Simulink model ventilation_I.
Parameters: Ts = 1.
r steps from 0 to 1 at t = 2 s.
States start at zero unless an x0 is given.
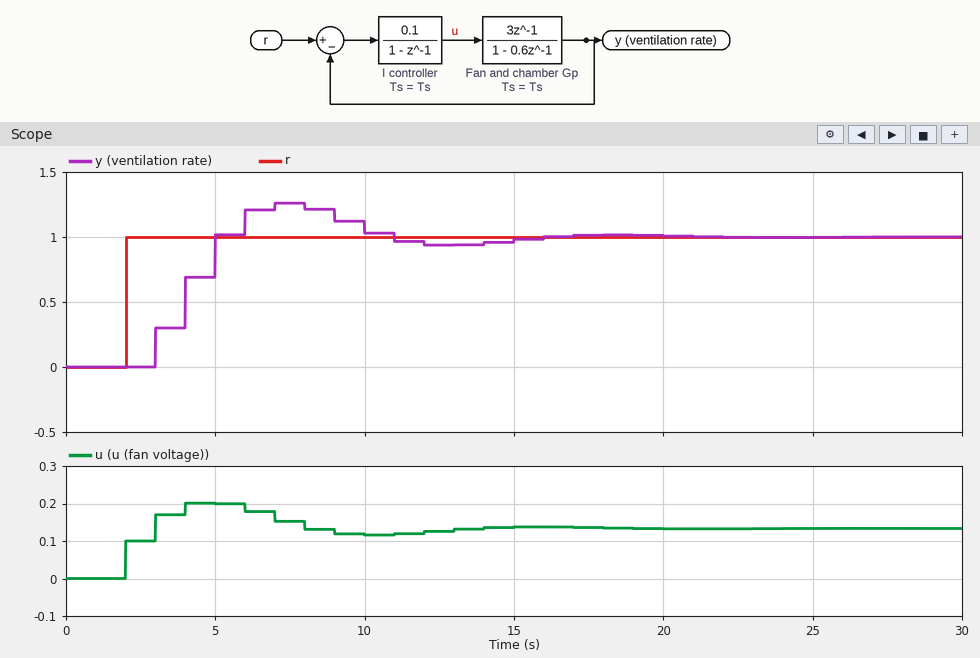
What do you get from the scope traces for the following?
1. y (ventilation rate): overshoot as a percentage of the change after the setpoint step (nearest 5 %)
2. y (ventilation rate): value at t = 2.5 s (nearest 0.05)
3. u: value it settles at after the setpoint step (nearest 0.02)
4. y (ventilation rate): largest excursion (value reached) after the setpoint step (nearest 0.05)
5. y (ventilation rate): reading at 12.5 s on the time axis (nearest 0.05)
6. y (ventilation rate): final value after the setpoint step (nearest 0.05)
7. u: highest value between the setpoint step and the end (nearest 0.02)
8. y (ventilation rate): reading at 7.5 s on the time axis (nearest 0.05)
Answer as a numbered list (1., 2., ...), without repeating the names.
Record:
1. 25 %
2. 0.00
3. 0.14
4. 1.25
5. 0.95
6. 1.00
7. 0.20
8. 1.25
